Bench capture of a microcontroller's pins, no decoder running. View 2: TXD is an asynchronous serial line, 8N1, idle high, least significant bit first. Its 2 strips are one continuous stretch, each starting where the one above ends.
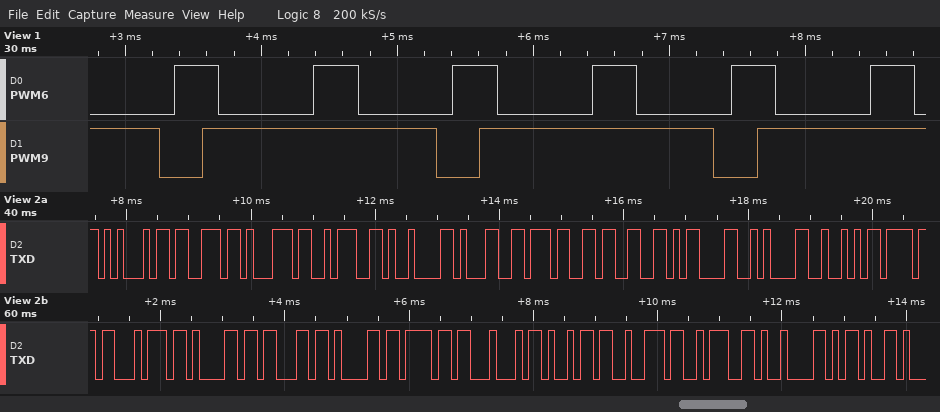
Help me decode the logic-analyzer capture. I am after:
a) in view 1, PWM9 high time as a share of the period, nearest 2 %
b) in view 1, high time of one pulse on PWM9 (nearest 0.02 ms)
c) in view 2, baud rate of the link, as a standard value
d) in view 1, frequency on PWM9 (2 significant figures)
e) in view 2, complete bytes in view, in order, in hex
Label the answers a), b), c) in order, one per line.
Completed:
a) 84 %
b) 1.72 ms
c) 9600 baud
d) 490 Hz
e) 45 73 71 3A 09 31 37 33 0D 0A 52 6F 74 61 63 61 6F 44 69 72 3A 09 2D
